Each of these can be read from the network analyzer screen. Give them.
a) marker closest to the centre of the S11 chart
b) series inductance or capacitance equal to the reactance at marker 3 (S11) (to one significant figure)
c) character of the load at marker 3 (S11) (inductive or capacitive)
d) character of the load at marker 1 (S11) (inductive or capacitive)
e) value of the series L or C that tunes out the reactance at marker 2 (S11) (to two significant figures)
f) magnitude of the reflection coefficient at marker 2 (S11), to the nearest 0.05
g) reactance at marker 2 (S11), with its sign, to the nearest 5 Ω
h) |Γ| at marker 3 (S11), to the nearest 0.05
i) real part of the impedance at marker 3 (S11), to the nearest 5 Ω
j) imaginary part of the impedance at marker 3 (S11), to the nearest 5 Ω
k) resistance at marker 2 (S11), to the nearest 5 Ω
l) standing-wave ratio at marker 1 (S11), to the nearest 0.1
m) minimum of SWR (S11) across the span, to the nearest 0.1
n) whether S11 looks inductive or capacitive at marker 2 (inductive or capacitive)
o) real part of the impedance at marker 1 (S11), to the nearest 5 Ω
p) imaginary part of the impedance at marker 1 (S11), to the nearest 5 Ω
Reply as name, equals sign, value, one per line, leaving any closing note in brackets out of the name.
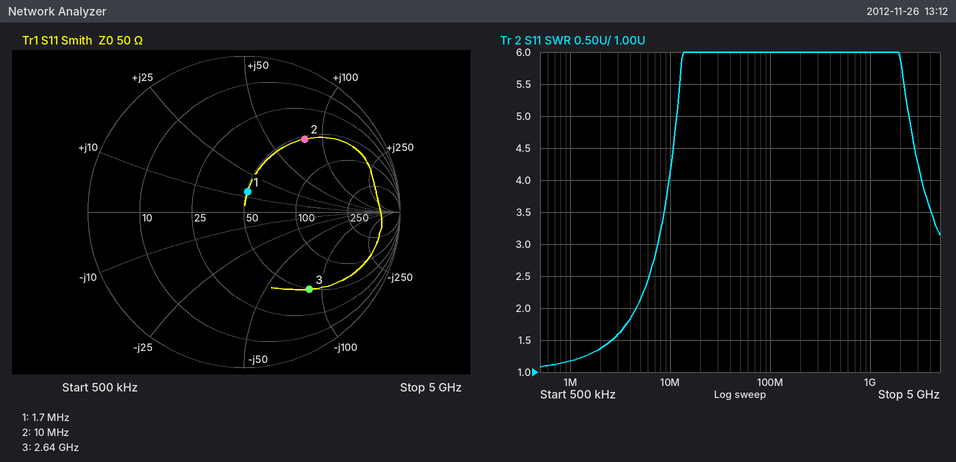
marker closest to the centre of the S11 chart = marker 1
series inductance or capacitance equal to the reactance at marker 3 (S11) = 700 fF
character of the load at marker 3 (S11) = capacitive
character of the load at marker 1 (S11) = inductive
value of the series L or C that tunes out the reactance at marker 2 (S11) = 200 pF
magnitude of the reflection coefficient at marker 2 (S11), to the nearest 0.05 = 0.60
reactance at marker 2 (S11), with its sign, to the nearest 5 Ω = +80 Ω
|Γ| at marker 3 (S11), to the nearest 0.05 = 0.65
real part of the impedance at marker 3 (S11), to the nearest 5 Ω = 50 Ω
imaginary part of the impedance at marker 3 (S11), to the nearest 5 Ω = -85 Ω
resistance at marker 2 (S11), to the nearest 5 Ω = 55 Ω
standing-wave ratio at marker 1 (S11), to the nearest 0.1 = 1.3
minimum of SWR (S11) across the span, to the nearest 0.1 = 1.1
whether S11 looks inductive or capacitive at marker 2 = inductive
real part of the impedance at marker 1 (S11), to the nearest 5 Ω = 50 Ω
imaginary part of the impedance at marker 1 (S11), to the nearest 5 Ω = +15 Ω
